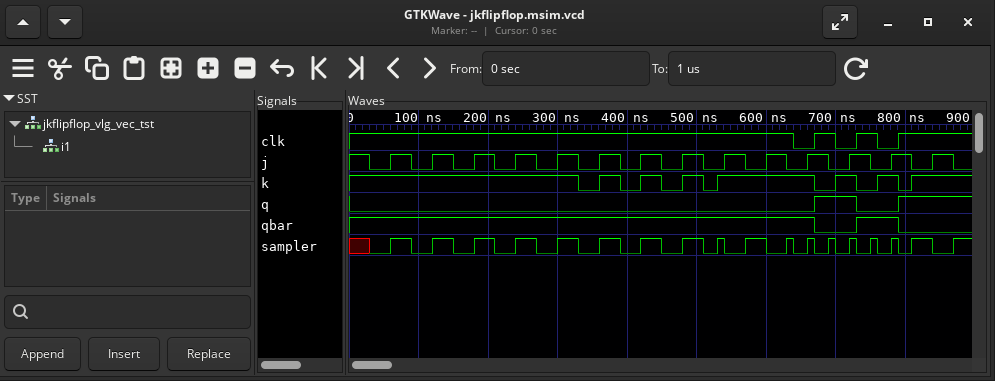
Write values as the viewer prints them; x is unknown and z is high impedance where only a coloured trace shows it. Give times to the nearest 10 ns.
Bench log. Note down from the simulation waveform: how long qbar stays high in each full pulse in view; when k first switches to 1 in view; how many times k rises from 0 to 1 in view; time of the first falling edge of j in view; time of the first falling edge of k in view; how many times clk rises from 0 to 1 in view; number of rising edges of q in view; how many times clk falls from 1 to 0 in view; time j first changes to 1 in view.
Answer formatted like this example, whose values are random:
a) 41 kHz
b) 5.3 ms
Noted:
a) 60 ns
b) 360 ns
c) 7
d) 30 ns
e) 330 ns
f) 3
g) 2
h) 3
i) 60 ns
